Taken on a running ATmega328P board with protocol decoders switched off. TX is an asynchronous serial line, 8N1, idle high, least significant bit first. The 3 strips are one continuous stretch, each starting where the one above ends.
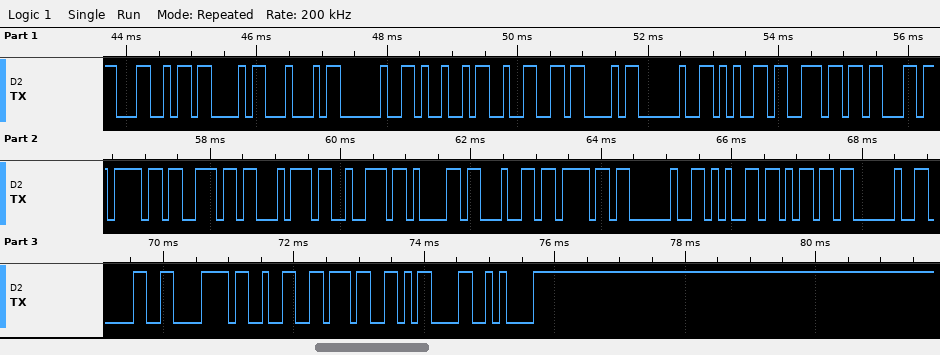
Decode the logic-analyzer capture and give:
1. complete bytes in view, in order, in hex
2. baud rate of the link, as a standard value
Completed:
4C 43 44 20 49 32 43 20 65 6E 63 6F 6E 74 72 61 64 6F 20 65 6D 20 30 78 32 37 0D 0A
9600 baud
